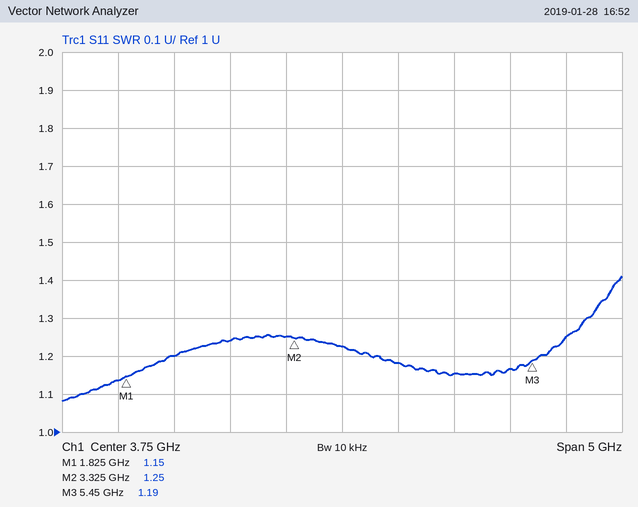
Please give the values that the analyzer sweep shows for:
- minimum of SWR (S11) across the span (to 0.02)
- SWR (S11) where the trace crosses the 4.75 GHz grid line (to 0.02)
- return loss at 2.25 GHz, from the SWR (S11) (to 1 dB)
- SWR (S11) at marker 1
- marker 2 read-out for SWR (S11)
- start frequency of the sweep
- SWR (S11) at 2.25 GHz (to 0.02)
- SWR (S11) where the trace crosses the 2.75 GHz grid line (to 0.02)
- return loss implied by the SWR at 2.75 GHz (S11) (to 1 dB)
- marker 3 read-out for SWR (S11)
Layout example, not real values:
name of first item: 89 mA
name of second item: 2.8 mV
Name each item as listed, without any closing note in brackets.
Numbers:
minimum of SWR (S11) across the span: 1.08
SWR (S11) where the trace crosses the 4.75 GHz grid line: 1.16
return loss at 2.25 GHz, from the SWR (S11): 21 dB
SWR (S11) at marker 1: 1.15
marker 2 read-out for SWR: 1.25
start frequency of the sweep: 1.25 GHz
SWR (S11) at 2.25 GHz: 1.20
SWR (S11) where the trace crosses the 2.75 GHz grid line: 1.24
return loss implied by the SWR at 2.75 GHz (S11): 19 dB
marker 3 read-out for SWR: 1.19
